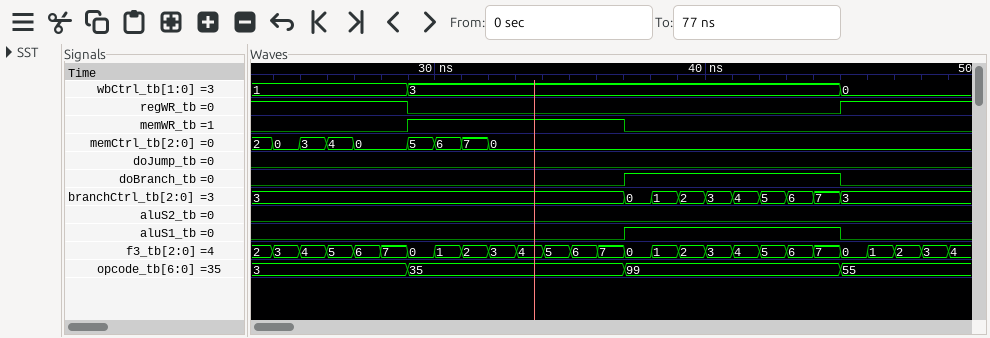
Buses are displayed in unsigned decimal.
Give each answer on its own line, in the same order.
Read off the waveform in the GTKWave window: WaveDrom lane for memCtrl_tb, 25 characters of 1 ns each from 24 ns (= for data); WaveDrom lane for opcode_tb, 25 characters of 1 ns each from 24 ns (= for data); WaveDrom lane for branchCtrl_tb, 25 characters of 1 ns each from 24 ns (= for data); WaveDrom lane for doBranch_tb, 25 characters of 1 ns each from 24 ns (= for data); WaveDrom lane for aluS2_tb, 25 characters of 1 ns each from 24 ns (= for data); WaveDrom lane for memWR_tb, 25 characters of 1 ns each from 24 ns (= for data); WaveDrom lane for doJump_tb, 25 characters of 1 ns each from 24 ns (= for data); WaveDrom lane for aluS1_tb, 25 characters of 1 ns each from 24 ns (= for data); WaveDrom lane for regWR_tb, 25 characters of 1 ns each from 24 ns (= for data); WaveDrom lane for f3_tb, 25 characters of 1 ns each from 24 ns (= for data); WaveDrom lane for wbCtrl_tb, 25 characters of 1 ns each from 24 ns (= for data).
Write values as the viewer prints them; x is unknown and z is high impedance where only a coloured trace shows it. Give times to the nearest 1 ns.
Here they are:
{name: 'memCtrl_tb', wave: '====.====................', data: '0 3 4 0 5 6 7 0'}
{name: 'opcode_tb', wave: '=....=.......=.......=...', data: '3 35 99 55'}
{name: 'branchCtrl_tb', wave: '=............=========...', data: '3 0 1 2 3 4 5 6 7 3'}
{name: 'doBranch_tb', wave: '0............1.......0...'}
{name: 'aluS2_tb', wave: '0........................'}
{name: 'memWR_tb', wave: '0....1.......0...........'}
{name: 'doJump_tb', wave: '0........................'}
{name: 'aluS1_tb', wave: '0............1.......0...'}
{name: 'regWR_tb', wave: '1....0...............1...'}
{name: 'f3_tb', wave: '=========================', data: '3 4 5 6 7 0 1 2 3 4 5 6 7 0 1 2 3 4 5 6 7 0 1 2 3'}
{name: 'wbCtrl_tb', wave: '=....=...............=...', data: '1 3 0'}
